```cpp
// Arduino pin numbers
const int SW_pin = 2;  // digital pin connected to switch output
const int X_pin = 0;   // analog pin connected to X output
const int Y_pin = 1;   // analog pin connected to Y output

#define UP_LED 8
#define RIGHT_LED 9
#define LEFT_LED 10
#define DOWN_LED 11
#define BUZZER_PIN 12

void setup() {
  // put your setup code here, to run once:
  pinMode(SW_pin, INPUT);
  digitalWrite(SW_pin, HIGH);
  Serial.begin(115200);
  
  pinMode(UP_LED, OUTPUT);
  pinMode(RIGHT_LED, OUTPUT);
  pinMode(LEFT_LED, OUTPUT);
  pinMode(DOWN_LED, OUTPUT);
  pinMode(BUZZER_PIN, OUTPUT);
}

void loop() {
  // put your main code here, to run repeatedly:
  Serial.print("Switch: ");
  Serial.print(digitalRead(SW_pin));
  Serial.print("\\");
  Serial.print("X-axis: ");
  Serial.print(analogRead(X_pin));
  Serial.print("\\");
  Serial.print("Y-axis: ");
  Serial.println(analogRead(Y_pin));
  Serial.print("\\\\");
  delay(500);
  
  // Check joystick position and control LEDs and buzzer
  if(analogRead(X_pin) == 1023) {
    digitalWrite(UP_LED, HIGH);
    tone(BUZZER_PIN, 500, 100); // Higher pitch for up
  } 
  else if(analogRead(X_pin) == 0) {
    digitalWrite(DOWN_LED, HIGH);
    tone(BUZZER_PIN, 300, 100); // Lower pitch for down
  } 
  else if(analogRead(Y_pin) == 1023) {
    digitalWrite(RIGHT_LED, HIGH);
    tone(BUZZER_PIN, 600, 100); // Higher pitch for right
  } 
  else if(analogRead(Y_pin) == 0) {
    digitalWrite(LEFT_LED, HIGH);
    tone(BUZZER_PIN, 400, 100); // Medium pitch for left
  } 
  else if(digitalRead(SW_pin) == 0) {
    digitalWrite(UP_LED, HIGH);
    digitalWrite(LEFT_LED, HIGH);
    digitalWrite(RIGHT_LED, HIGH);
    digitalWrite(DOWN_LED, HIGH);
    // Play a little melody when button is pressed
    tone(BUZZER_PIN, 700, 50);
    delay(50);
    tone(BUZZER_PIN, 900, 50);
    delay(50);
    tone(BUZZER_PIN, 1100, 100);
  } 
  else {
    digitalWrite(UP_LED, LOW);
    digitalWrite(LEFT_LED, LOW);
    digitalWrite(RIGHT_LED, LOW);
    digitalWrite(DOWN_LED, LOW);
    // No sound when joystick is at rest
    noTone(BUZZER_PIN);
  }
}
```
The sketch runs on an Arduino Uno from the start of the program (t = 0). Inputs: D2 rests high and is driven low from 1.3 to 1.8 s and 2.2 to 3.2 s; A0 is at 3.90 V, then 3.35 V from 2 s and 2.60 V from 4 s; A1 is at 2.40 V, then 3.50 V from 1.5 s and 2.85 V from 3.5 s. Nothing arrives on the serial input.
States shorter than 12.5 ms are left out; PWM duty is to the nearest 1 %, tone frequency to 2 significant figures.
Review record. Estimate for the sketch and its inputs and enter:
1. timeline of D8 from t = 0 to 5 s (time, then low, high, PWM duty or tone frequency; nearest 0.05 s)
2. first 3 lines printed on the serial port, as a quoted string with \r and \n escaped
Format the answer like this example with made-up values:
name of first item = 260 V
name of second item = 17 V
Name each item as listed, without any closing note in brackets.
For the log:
timeline of D8 from t = 0 to 5 s = 0 s low; 1.5 s high; 2.1 s low; 2.6 s high; 3.2 s low
first 3 lines printed on the serial port, as a quoted string with \r and \n escaped = "Switch: 1\\X-axis: 798\\Y-axis: 491\r\n\\\\Switch: 1\\X-axis: 798\\Y-axis: 491\r\n\\\\Switch: 1\\X-axis: 798\\Y-axis: 491\r\n"
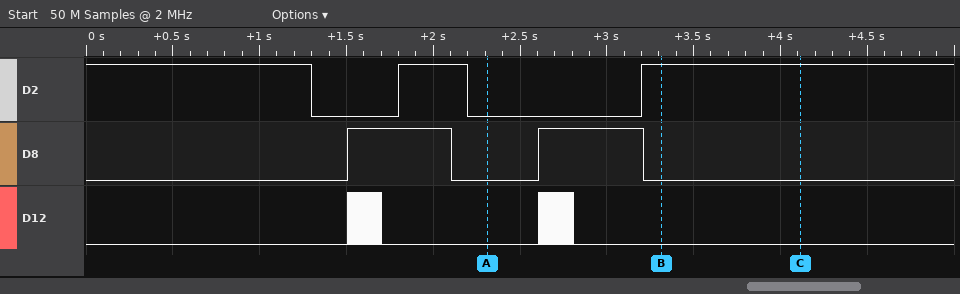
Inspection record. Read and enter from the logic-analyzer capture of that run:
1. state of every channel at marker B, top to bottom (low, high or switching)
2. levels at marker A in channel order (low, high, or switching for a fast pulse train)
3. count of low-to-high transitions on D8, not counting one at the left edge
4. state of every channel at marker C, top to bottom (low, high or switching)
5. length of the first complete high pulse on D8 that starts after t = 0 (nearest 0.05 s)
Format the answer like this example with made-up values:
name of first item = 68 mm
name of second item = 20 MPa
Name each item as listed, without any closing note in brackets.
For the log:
state of every channel at marker B, top to bottom = D2 high, D8 low, D12 low
levels at marker A in channel order = D2 low, D8 low, D12 low
count of low-to-high transitions on D8, not counting one at the left edge = 2
state of every channel at marker C, top to bottom = D2 high, D8 low, D12 low
length of the first complete high pulse on D8 that starts after t = 0 = 0.60 s
